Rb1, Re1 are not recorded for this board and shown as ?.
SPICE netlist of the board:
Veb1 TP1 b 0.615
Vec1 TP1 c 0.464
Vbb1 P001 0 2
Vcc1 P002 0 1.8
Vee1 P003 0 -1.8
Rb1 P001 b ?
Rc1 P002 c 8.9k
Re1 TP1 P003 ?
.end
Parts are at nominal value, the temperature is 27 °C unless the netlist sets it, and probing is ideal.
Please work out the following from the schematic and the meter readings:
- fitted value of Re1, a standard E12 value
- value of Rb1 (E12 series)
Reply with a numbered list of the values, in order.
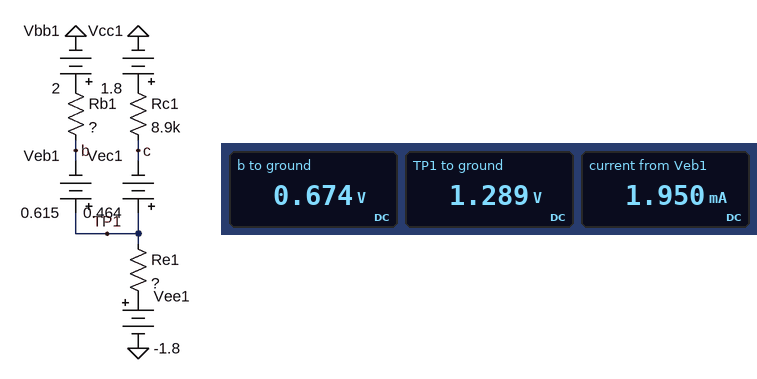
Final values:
1. 1.5 kΩ
2. 680 Ω
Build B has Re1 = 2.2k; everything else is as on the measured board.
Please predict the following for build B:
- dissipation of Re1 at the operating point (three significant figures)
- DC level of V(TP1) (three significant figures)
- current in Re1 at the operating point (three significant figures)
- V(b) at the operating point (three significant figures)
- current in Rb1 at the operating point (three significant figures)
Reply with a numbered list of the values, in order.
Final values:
1. 5.29 mW
2. 1.61 V
3. 1.55 mA
4. 996 mV
5. 1.48 mA
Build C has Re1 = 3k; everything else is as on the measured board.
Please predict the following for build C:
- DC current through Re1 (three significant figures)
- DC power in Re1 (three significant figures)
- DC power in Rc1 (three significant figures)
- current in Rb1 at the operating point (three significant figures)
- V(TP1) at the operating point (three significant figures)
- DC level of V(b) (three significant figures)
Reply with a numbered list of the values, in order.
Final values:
1. 1.21 mA
2. 4.38 mW
3. 21.5 µW
4. 1.16 mA
5. 1.83 V
6. 1.21 V
